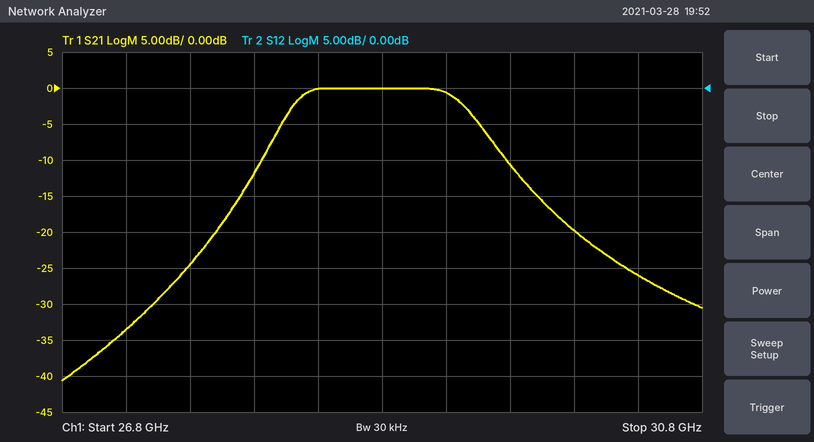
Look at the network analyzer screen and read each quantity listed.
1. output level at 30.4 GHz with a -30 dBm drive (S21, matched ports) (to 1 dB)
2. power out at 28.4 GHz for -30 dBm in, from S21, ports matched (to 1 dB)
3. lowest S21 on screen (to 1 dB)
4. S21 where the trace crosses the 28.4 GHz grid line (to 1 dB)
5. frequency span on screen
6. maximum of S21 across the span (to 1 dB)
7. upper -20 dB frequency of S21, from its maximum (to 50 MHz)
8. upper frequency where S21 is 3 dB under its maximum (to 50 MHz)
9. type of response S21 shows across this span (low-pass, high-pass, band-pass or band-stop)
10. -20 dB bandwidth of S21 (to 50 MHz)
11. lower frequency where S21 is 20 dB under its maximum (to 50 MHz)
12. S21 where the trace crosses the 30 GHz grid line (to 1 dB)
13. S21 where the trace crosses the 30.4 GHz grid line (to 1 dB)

-56 dBm
-30 dBm
-41 dB
0 dB
4 GHz
0 dB
30.00 GHz
29.35 GHz
band-pass
2.25 GHz
27.75 GHz
-20 dB
-26 dB
